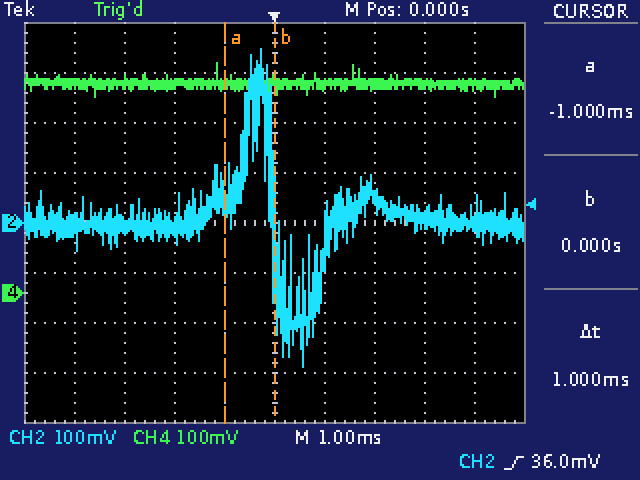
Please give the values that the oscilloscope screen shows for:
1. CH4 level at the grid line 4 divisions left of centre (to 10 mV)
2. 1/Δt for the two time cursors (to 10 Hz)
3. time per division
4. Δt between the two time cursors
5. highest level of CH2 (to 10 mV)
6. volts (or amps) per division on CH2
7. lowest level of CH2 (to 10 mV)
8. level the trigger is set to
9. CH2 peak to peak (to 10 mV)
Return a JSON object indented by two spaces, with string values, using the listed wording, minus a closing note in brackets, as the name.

{
  "CH4 level at the grid line 4 divisions left of centre": "420 mV",
  "1/Δt for the two time cursors": "1.00 kHz",
  "time per division": "1 ms",
  "Δt between the two time cursors": "1 ms",
  "highest level of CH2": "350 mV",
  "volts (or amps) per division on CH2": "100 mV",
  "lowest level of CH2": "-290 mV",
  "level the trigger is set to": "36.0 mV",
  "CH2 peak to peak": "640 mV"
}
